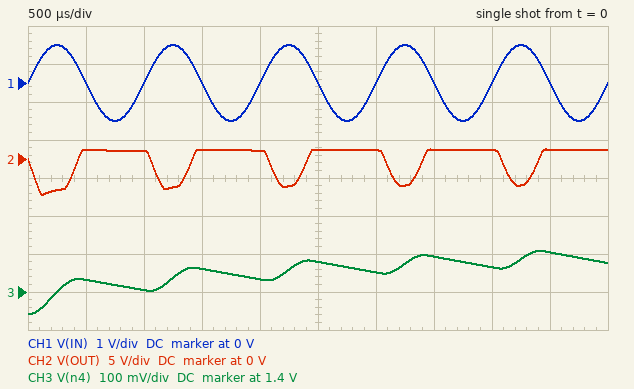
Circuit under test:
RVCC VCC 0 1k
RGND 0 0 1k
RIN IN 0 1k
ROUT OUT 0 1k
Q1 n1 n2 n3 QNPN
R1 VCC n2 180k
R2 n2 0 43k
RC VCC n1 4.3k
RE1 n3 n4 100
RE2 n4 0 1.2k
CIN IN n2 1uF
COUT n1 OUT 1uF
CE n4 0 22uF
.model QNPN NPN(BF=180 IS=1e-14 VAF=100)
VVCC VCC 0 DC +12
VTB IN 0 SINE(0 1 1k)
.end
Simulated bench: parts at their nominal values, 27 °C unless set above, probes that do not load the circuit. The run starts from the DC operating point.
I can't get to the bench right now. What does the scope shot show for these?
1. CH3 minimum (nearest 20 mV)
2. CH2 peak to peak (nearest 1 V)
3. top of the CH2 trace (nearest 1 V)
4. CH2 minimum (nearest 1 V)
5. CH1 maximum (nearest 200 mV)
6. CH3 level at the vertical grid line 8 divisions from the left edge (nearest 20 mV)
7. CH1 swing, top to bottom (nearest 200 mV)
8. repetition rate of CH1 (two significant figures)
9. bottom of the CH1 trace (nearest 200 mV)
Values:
1.34 V
6 V
1 V
-5 V
1.0 V
1.46 V
2.0 V
1.0 kHz
-1.0 V
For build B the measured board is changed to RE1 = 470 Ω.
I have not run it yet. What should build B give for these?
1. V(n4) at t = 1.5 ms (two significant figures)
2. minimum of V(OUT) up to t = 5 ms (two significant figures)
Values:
1.1 V
-1.6 V
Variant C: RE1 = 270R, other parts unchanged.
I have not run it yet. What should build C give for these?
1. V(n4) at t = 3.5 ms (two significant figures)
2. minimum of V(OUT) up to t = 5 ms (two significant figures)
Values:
1.3 V
-2.7 V
